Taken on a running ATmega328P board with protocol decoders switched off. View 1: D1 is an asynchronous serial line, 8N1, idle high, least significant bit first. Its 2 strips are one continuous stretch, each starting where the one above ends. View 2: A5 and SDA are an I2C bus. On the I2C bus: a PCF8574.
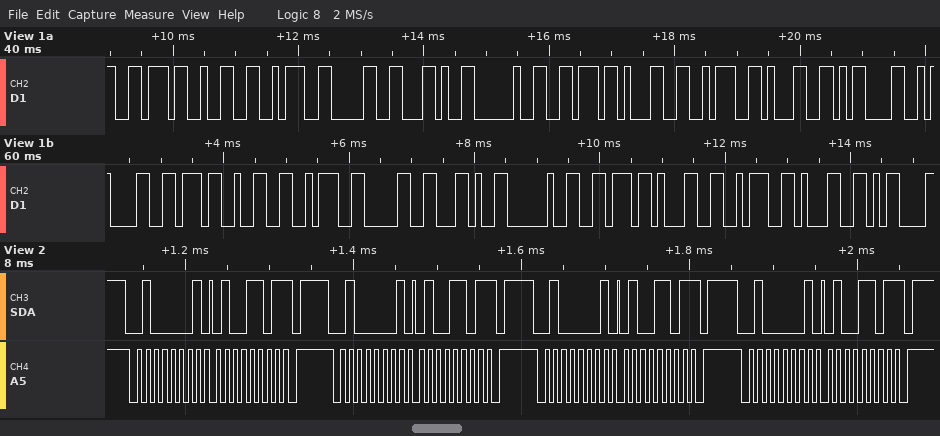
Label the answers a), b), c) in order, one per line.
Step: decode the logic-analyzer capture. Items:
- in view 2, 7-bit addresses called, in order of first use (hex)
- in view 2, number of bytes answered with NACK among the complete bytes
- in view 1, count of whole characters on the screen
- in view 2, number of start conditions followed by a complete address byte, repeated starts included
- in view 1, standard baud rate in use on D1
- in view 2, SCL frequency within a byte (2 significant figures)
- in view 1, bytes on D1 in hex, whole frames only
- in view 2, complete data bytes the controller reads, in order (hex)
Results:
a) 0x20
b) 4
c) 23
d) 4
e) 9600 baud
f) 100 kHz
g) 0x76 0x32 0x3A 0x30 0x2C 0x20 0x76 0x31 0x3A 0x31 0x0D 0x0A 0x76 0x32 0x3A 0x30 0x2C 0x20 0x76 0x31 0x3A 0x31 0x0D
h) 4D 4D 4D 4D
